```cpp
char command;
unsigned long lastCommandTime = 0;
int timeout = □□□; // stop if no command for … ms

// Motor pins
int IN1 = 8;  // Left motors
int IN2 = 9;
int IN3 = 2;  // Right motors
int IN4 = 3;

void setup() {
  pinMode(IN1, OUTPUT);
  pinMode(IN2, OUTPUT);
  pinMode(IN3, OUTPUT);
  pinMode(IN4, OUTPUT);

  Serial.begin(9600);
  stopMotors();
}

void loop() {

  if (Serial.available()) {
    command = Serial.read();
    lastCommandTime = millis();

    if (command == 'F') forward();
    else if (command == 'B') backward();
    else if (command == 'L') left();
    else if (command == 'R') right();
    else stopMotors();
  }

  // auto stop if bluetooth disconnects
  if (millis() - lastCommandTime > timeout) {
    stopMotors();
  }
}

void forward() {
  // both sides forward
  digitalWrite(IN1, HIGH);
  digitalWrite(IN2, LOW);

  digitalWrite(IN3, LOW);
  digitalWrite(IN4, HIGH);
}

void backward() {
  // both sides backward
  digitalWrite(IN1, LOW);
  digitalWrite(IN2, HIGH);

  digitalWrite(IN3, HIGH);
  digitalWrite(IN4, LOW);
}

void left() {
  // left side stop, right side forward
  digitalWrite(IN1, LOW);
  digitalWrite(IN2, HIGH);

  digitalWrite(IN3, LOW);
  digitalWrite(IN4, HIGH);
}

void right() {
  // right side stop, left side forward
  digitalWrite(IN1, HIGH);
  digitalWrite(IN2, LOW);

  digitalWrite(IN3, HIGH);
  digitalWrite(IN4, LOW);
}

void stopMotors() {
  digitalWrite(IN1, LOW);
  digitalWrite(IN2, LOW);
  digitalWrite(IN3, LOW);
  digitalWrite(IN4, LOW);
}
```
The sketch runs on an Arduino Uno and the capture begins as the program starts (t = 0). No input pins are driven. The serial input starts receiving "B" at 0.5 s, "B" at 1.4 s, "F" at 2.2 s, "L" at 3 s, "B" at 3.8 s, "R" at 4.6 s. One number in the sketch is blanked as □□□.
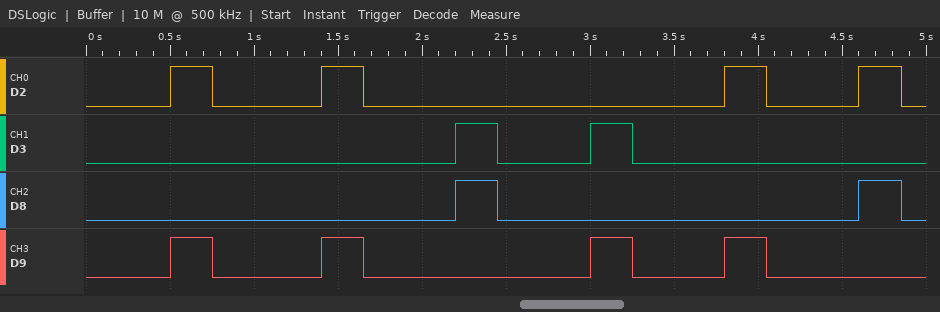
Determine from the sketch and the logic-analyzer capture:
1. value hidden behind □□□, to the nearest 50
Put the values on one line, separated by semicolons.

250
